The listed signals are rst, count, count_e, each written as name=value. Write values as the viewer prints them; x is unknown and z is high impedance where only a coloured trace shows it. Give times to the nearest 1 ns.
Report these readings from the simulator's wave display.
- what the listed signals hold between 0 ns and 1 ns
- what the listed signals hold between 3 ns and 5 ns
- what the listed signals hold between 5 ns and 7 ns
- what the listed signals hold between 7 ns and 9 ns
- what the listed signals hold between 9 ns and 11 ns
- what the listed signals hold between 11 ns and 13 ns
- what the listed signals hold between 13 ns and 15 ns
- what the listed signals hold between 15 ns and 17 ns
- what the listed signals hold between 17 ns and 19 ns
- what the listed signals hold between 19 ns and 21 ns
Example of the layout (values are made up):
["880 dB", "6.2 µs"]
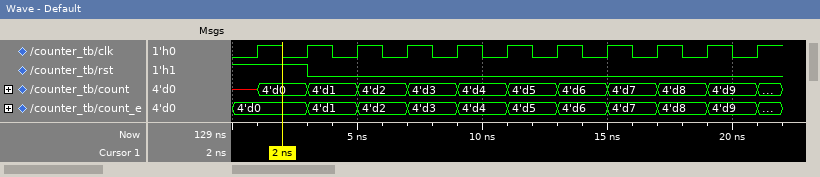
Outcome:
["rst=1, count=x, count_e=4'd0", "rst=0, count=4'd1, count_e=4'd1", "rst=0, count=4'd2, count_e=4'd2", "rst=0, count=4'd3, count_e=4'd3", "rst=0, count=4'd4, count_e=4'd4", "rst=0, count=4'd5, count_e=4'd5", "rst=0, count=4'd6, count_e=4'd6", "rst=0, count=4'd7, count_e=4'd7", "rst=0, count=4'd8, count_e=4'd8", "rst=0, count=4'd9, count_e=4'd9"]
